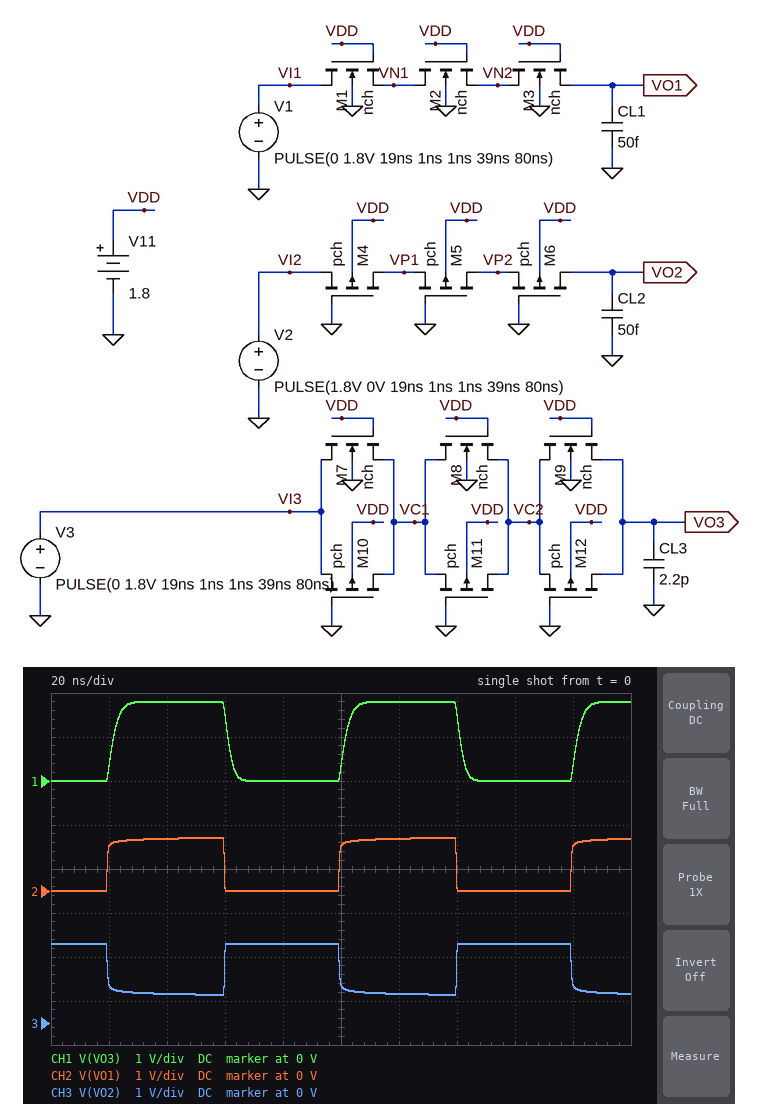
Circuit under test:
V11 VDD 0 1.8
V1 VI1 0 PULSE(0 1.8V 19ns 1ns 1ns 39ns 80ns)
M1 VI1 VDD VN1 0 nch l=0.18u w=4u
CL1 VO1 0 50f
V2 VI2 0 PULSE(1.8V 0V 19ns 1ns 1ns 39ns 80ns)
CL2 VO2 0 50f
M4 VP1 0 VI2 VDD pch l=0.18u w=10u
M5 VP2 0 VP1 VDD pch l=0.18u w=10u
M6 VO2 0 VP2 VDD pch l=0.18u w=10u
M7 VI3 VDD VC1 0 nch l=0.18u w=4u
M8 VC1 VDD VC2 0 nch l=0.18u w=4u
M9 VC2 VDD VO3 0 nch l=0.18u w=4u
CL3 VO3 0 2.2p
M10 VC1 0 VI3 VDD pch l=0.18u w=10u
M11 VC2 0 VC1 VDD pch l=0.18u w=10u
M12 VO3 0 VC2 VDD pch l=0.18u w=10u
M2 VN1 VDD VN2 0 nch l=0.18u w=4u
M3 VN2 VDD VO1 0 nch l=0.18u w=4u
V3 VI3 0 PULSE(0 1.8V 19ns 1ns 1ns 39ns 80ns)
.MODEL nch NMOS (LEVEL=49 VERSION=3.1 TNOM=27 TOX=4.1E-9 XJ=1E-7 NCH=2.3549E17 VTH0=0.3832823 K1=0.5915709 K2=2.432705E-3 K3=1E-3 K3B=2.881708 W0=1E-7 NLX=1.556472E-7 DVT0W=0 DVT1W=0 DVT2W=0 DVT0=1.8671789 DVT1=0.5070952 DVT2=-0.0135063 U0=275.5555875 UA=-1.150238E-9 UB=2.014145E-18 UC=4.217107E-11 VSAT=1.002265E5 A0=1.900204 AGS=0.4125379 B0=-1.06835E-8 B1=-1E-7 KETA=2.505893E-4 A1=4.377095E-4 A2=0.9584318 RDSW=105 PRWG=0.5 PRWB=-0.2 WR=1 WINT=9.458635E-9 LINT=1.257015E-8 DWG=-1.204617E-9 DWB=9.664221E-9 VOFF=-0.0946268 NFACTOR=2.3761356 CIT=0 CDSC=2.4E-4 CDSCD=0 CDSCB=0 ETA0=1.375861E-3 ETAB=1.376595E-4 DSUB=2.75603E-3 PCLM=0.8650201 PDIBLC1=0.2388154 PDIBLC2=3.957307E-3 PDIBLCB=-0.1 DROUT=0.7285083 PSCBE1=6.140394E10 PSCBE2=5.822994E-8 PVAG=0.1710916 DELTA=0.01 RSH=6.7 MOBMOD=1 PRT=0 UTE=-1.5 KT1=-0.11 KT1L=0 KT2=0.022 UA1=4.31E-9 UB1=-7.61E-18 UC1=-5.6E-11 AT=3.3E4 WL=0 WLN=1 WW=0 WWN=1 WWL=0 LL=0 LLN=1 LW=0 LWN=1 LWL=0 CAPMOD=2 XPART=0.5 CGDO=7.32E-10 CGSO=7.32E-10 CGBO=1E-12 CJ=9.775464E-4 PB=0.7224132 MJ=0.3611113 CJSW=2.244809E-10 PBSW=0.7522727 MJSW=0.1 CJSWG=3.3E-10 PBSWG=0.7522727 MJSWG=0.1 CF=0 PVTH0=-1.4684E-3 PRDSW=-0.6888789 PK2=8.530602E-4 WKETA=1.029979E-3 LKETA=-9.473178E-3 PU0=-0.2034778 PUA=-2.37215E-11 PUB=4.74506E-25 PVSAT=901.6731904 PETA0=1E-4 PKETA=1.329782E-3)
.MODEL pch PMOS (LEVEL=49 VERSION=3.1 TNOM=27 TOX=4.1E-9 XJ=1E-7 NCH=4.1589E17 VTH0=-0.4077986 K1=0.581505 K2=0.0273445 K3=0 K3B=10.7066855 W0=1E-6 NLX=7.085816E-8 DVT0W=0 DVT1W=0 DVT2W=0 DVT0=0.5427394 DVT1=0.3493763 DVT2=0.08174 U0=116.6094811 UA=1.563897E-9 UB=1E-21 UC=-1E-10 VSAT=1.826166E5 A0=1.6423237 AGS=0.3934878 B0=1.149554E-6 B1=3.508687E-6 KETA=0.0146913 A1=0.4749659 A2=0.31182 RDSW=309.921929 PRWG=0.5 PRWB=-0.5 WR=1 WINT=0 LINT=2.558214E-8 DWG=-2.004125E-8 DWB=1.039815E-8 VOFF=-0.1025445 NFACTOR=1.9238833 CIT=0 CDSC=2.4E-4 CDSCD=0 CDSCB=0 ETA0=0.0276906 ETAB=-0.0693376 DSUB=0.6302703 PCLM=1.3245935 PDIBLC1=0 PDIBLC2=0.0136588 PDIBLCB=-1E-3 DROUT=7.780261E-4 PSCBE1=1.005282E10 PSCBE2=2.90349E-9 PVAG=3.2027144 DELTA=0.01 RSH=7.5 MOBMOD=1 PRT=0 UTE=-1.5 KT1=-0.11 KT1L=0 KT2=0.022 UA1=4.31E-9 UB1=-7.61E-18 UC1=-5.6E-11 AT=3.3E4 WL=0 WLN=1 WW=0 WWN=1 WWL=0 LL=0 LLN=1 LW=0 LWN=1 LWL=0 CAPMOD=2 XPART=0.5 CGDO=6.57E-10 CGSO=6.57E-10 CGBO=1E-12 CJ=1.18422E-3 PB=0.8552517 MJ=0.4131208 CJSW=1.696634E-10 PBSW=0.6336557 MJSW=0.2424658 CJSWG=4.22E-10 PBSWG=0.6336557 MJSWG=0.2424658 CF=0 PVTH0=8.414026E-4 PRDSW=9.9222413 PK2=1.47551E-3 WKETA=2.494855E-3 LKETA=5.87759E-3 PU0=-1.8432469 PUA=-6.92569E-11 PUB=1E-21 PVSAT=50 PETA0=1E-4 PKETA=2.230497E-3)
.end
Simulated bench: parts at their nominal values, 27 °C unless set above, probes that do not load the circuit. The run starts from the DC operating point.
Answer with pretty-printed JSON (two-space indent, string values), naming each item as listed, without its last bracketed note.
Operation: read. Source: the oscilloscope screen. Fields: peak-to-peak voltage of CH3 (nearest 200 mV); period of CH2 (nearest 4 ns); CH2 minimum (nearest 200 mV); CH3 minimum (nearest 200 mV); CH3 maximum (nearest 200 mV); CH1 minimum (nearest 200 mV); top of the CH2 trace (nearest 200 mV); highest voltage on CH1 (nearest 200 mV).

{
  "peak-to-peak voltage of CH3": "1.2 V",
  "period of CH2": "80 ns",
  "CH2 minimum": "0 V",
  "CH3 minimum": "600 mV",
  "CH3 maximum": "1.8 V",
  "CH1 minimum": "0 V",
  "top of the CH2 trace": "1.2 V",
  "highest voltage on CH1": "1.8 V"
}
